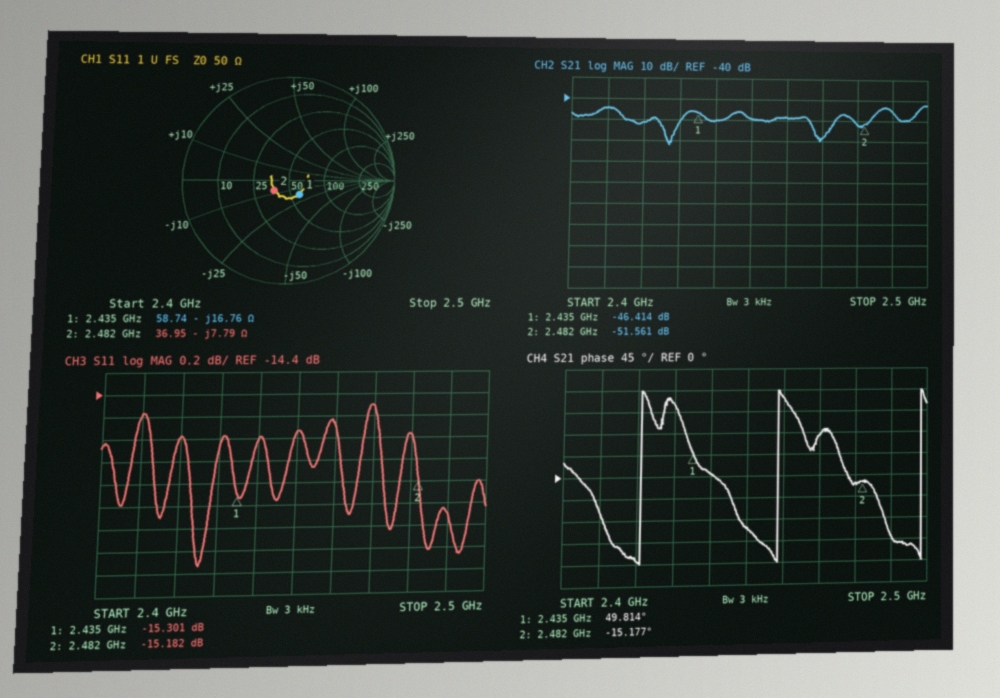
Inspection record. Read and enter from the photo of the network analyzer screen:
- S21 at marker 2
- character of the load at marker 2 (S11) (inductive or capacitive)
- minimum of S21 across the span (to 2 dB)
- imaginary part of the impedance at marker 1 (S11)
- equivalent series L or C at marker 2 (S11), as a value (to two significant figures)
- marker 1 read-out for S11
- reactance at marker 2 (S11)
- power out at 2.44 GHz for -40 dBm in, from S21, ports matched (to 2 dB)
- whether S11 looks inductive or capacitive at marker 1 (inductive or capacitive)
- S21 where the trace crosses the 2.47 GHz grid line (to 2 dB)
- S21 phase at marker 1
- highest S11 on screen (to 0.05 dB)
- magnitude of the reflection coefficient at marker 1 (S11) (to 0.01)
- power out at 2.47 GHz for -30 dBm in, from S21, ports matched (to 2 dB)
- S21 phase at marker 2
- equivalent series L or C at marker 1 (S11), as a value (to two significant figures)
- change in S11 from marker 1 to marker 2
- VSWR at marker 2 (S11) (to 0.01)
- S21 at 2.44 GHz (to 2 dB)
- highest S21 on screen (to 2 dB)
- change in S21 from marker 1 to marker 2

-51.561 dB
capacitive
-62 dB
-16.76 Ω
8.2 pF
-15.301 dB
-7.79 Ω
-90 dBm
capacitive
-58 dB
49.814°
-14.50 dB
0.17
-88 dBm
-15.177°
3.9 pF
0.119 dB
1.42
-50 dB
-42 dB
-5.147 dB
